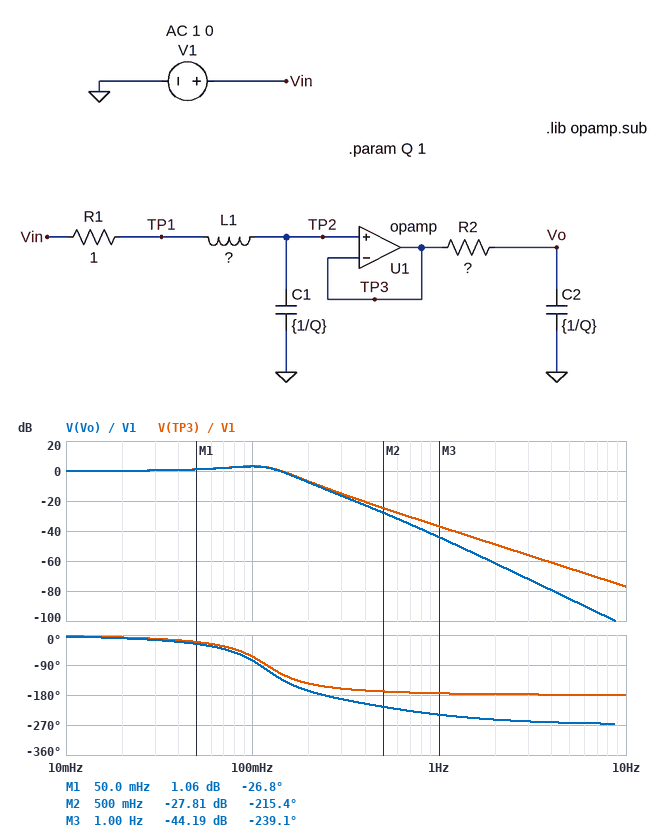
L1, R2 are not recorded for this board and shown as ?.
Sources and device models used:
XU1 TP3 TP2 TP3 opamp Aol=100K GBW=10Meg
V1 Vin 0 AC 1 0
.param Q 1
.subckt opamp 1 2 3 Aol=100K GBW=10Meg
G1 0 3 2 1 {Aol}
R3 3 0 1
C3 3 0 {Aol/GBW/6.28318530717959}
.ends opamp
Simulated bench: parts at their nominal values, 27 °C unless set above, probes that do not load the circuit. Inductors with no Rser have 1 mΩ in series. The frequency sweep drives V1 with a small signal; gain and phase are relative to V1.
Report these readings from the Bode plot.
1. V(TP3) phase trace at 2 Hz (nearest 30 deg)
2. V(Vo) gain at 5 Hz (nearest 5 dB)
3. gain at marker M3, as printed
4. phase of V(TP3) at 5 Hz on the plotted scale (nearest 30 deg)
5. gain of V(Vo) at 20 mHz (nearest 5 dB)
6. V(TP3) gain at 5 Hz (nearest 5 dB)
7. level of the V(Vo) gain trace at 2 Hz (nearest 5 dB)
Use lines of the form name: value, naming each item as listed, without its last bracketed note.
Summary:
V(TP3) phase trace at 2 Hz: -180 deg
V(Vo) gain at 5 Hz: -85 dB
gain at marker M3, as printed: -44.19 dB
phase of V(TP3) at 5 Hz on the plotted scale: -180 deg
gain of V(Vo) at 20 mHz: 0 dB
V(TP3) gain at 5 Hz: -65 dB
level of the V(Vo) gain trace at 2 Hz: -60 dB
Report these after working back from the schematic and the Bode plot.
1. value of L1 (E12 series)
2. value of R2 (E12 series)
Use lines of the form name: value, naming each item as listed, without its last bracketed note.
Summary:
value of L1: 1.8 H
value of R2: 0.33 Ω
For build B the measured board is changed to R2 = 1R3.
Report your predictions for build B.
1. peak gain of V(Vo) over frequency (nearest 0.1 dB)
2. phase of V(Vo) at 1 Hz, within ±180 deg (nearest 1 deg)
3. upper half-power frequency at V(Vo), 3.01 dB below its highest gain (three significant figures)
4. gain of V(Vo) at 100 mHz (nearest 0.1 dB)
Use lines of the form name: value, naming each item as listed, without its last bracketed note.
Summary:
peak gain of V(Vo) over frequency: 1.1 dB
phase of V(Vo) at 1 Hz, within ±180 deg: 102 deg
upper half-power frequency at V(Vo), 3.01 dB below its highest gain: 131 mHz
gain of V(Vo) at 100 mHz: 1.0 dB
